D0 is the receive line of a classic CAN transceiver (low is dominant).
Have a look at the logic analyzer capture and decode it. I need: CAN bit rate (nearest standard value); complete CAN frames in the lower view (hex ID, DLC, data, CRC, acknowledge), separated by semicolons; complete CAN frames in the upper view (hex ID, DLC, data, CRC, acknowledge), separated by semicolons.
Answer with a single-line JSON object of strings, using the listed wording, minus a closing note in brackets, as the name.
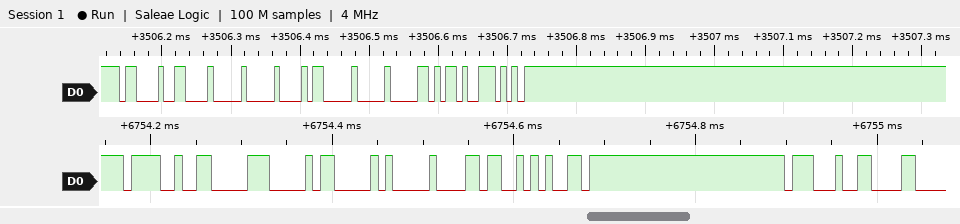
{"CAN bit rate": "125 kbit/s", "complete CAN frames in the lower view (hex ID, DLC, data, CRC, acknowledge), separated by semicolons": "ID 793, DLC 3, data 03 02 00, CRC 6CA9, ACK", "complete CAN frames in the upper view (hex ID, DLC, data, CRC, acknowledge), separated by semicolons": "ID 613, DLC 4, data 00 0B 00 01, CRC 2D3A, ACK"}
